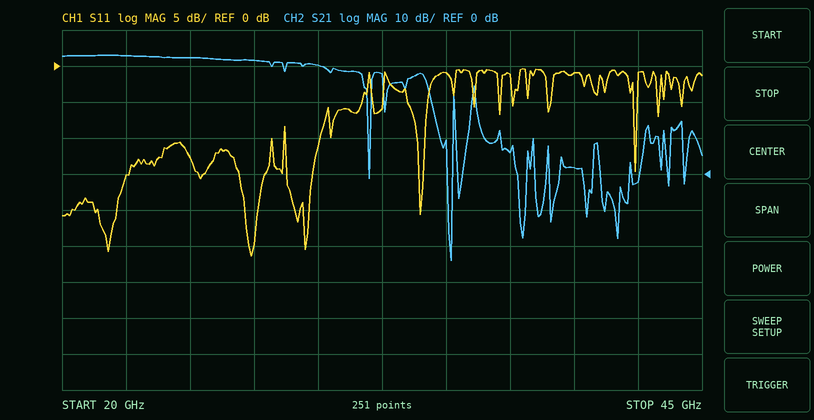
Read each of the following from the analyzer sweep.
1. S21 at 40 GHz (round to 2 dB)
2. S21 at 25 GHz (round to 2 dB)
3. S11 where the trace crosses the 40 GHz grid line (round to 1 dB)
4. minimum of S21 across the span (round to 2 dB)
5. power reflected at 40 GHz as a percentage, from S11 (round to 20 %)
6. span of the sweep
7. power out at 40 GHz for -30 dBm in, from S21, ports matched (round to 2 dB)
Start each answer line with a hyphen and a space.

- 2 dB
- 32 dB
- -1 dB
- -24 dB
- 80 %
- 25 GHz
- -28 dBm
